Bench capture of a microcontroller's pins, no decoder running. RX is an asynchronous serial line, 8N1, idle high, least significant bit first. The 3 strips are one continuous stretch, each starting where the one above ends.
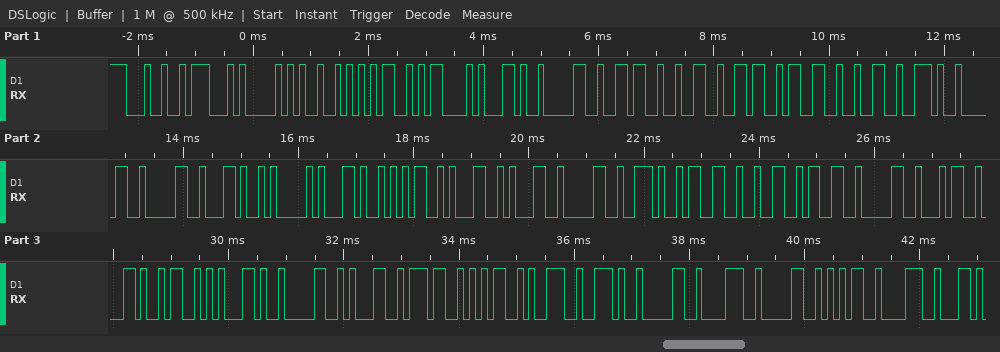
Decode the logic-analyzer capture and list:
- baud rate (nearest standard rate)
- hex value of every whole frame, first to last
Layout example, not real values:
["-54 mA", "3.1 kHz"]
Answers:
["9600 baud", "24 47 50 52 4D 43 2C 30 36 32 36 33 32 2E 30 30 2C 41 2C 35 31 31 30 2E 33 32 33 30 34 2C 53 2C 30 31 37 35 39 2E 30 38 30 35 38"]
